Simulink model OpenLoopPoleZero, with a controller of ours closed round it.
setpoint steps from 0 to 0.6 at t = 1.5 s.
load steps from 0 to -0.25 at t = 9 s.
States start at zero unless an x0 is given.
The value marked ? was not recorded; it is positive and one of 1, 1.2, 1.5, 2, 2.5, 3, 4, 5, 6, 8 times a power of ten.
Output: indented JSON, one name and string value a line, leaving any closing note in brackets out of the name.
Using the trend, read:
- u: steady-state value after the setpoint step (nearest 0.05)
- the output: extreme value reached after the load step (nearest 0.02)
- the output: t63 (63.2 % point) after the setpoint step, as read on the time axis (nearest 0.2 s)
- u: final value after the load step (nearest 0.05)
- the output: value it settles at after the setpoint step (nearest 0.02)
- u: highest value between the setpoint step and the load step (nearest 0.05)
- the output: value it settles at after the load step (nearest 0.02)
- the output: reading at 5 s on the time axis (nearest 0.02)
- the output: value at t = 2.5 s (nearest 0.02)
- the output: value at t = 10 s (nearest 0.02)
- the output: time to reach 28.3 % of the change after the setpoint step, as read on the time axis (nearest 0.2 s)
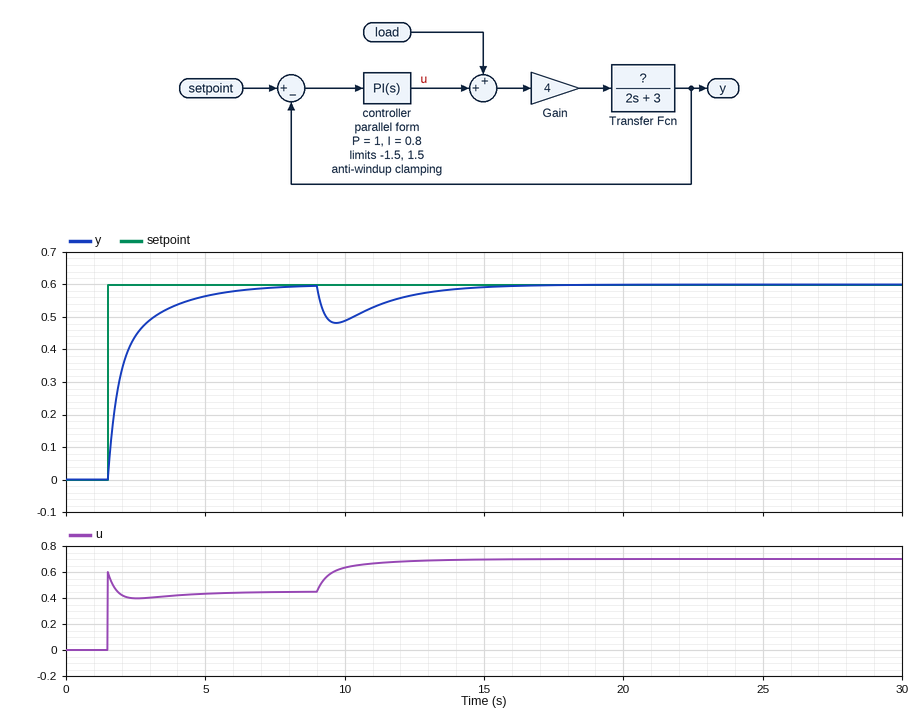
{
  "u: steady-state value after the setpoint step": "0.45",
  "the output: extreme value reached after the load step": "0.48",
  "the output: t63 (63.2 % point) after the setpoint step, as read on the time axis": "2.2 s",
  "u: final value after the load step": "0.70",
  "the output: value it settles at after the setpoint step": "0.60",
  "u: highest value between the setpoint step and the load step": "0.60",
  "the output: value it settles at after the load step": "0.60",
  "the output: reading at 5 s on the time axis": "0.56",
  "the output: value at t = 2.5 s": "0.44",
  "the output: value at t = 10 s": "0.48",
  "the output: time to reach 28.3 % of the change after the setpoint step, as read on the time axis": "1.6 s"
}
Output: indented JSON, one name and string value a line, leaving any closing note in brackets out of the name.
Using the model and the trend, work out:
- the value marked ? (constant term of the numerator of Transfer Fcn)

{
  "the value marked ?": "1"
}
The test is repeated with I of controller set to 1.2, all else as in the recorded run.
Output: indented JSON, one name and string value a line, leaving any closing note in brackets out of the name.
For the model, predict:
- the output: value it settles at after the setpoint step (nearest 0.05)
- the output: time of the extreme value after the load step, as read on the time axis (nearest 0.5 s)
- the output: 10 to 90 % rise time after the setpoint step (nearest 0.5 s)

{
  "the output: value it settles at after the setpoint step": "0.60",
  "the output: time of the extreme value after the load step, as read on the time axis": "9.5 s",
  "the output: 10 to 90 % rise time after the setpoint step": "1.5 s"
}
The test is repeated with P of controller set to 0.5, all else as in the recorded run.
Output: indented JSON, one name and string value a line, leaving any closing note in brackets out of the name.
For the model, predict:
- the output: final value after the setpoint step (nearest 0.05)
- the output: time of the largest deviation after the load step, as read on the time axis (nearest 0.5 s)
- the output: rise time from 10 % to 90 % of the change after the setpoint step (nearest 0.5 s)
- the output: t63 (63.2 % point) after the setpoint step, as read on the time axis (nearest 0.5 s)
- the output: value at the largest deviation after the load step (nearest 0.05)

{
  "the output: final value after the setpoint step": "0.60",
  "the output: time of the largest deviation after the load step, as read on the time axis": "10.0 s",
  "the output: rise time from 10 % to 90 % of the change after the setpoint step": "2.0 s",
  "the output: t63 (63.2 % point) after the setpoint step, as read on the time axis": "2.5 s",
  "the output: value at the largest deviation after the load step": "0.45"
}
